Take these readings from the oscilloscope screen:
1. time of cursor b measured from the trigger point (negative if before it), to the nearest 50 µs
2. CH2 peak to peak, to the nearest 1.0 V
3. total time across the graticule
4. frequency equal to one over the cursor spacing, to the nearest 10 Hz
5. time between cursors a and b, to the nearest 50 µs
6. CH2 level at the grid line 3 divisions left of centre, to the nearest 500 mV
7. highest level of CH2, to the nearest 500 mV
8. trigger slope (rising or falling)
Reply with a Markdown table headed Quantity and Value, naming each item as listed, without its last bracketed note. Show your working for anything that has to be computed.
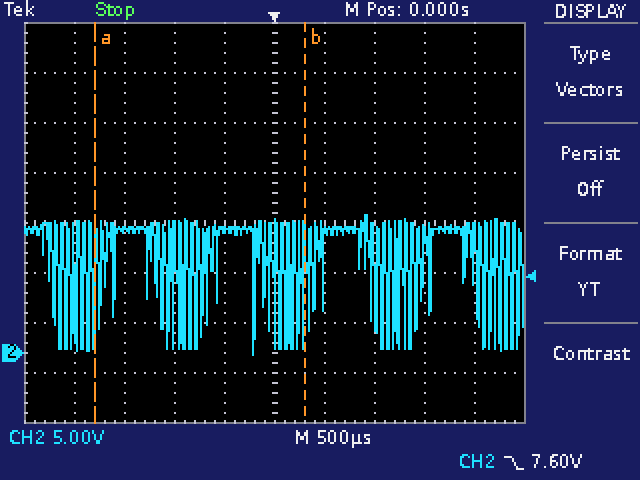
| Quantity | Value |
|---|---|
| time of cursor b measured from the trigger point (negative if before it), to the nearest 50 µs | +300 µs |
| CH2 peak to peak, to the nearest 1.0 V | 14.0 V |
| total time across the graticule | 5 ms |
| frequency equal to one over the cursor spacing, to the nearest 10 Hz | 1 / 2.10 ms ≈ 480 Hz |
| time between cursors a and b, to the nearest 50 µs | 2.10 ms |
| CH2 level at the grid line 3 divisions left of centre, to the nearest 500 mV | 12.5 V |
| highest level of CH2, to the nearest 500 mV | 14.0 V |
| trigger slope | falling |
